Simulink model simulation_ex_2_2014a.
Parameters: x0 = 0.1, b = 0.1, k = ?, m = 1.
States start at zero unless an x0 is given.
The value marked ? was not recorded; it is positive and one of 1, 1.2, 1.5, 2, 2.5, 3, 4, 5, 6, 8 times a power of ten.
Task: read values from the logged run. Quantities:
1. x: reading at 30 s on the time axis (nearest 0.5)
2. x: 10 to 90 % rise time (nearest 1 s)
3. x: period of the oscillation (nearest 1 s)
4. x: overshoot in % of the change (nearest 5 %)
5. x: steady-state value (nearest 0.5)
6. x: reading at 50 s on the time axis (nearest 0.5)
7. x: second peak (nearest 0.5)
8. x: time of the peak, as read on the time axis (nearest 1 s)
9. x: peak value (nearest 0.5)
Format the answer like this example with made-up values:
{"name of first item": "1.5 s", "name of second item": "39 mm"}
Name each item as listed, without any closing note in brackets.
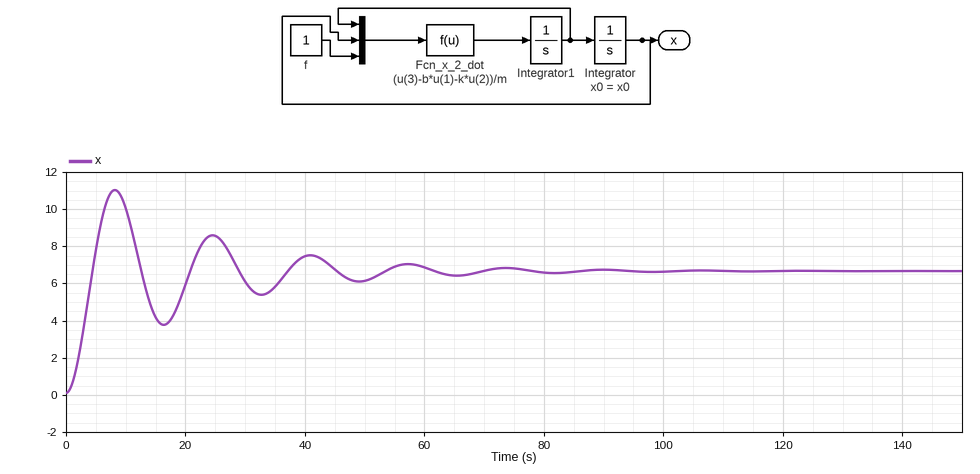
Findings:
{"x: reading at 30 s on the time axis": "6.0", "x: 10 to 90 % rise time": "3 s", "x: period of the oscillation": "16 s", "x: overshoot in % of the change": "65 %", "x: steady-state value": "6.5", "x: reading at 50 s on the time axis": "6.0", "x: second peak": "8.5", "x: time of the peak, as read on the time axis": "8 s", "x: peak value": "11.0"}
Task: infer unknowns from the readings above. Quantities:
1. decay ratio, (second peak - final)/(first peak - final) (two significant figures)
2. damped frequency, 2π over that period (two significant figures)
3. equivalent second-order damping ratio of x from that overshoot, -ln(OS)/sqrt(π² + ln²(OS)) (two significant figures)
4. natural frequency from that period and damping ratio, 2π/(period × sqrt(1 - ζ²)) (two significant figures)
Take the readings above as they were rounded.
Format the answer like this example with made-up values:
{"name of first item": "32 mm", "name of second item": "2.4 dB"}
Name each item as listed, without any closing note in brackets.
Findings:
{"decay ratio, (second peak - final)/(first peak - final)": "0.44", "damped frequency, 2π over that period": "0.39 rad/s", "equivalent second-order damping ratio of x from that overshoot, -ln(OS)/sqrt(π² + ln²(OS))": "0.14", "natural frequency from that period and damping ratio, 2π/(period × sqrt(1 - ζ²))": "0.40 rad/s"}
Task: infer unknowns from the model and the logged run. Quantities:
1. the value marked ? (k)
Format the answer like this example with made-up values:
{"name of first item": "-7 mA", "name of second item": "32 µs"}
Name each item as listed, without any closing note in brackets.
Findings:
{"the value marked ?": "0.15"}
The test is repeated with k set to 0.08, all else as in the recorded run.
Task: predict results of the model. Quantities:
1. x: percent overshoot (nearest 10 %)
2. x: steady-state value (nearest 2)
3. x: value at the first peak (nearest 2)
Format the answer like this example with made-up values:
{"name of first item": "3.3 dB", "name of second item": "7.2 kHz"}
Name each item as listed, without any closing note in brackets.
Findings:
{"x: percent overshoot": "60 %", "x: steady-state value": "12", "x: value at the first peak": "20"}
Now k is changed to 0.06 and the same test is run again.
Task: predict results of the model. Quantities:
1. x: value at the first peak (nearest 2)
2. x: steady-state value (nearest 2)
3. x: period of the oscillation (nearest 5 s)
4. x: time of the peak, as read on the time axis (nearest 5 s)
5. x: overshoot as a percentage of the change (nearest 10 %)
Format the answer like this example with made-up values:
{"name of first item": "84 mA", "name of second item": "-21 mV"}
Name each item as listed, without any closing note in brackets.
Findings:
{"x: value at the first peak": "26", "x: steady-state value": "16", "x: period of the oscillation": "25 s", "x: time of the peak, as read on the time axis": "15 s", "x: overshoot as a percentage of the change": "50 %"}
